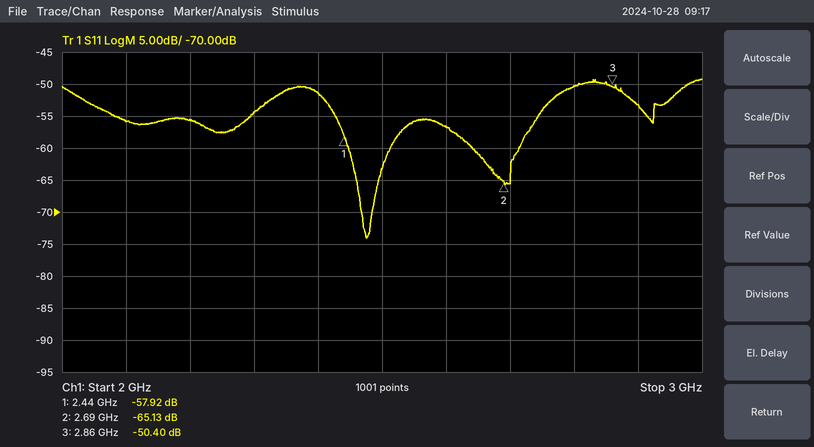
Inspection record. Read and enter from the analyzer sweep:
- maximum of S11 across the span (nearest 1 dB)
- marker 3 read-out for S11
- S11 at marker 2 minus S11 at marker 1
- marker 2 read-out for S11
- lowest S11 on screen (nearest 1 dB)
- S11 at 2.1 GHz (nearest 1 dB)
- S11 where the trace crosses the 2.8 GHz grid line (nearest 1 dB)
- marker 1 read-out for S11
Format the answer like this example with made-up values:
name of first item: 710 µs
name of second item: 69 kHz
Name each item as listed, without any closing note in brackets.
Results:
maximum of S11 across the span: -49 dB
marker 3 read-out for S11: -50.40 dB
S11 at marker 2 minus S11 at marker 1: -7.21 dB
marker 2 read-out for S11: -65.13 dB
lowest S11 on screen: -74 dB
S11 at 2.1 GHz: -56 dB
S11 where the trace crosses the 2.8 GHz grid line: -50 dB
marker 1 read-out for S11: -57.92 dB
